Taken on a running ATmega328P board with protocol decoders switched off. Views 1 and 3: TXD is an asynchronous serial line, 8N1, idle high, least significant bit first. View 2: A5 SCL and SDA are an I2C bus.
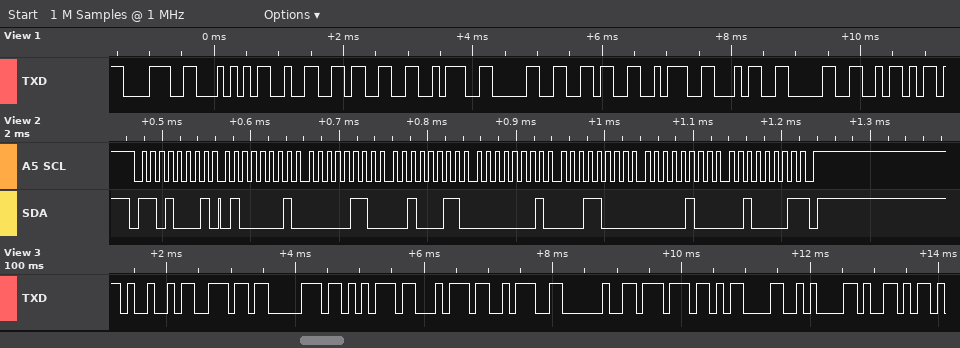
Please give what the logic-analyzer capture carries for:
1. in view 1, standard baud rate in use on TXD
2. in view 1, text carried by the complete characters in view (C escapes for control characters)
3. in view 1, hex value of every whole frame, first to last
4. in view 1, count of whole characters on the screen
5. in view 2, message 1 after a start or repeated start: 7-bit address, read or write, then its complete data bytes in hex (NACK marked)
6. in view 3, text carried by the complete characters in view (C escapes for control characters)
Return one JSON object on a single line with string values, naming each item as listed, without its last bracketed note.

{"in view 1, standard baud rate in use on TXD": "9600 baud", "in view 1, text carried by the complete characters in view": "\"8T23:06:40Z\"", "in view 1, hex value of every whole frame, first to last": "38 54 32 33 3A 30 36 3A 34 30 5A", "in view 1, count of whole characters on the screen": "11", "in view 2, message 1 after a start or repeated start: 7-bit address, read or write, then its complete data bytes in hex": "0x68 read: 41 06 23 01 18 04 21 NACK", "in view 3, text carried by the complete characters in view": "\"Input: w\\r\\nY\""}
